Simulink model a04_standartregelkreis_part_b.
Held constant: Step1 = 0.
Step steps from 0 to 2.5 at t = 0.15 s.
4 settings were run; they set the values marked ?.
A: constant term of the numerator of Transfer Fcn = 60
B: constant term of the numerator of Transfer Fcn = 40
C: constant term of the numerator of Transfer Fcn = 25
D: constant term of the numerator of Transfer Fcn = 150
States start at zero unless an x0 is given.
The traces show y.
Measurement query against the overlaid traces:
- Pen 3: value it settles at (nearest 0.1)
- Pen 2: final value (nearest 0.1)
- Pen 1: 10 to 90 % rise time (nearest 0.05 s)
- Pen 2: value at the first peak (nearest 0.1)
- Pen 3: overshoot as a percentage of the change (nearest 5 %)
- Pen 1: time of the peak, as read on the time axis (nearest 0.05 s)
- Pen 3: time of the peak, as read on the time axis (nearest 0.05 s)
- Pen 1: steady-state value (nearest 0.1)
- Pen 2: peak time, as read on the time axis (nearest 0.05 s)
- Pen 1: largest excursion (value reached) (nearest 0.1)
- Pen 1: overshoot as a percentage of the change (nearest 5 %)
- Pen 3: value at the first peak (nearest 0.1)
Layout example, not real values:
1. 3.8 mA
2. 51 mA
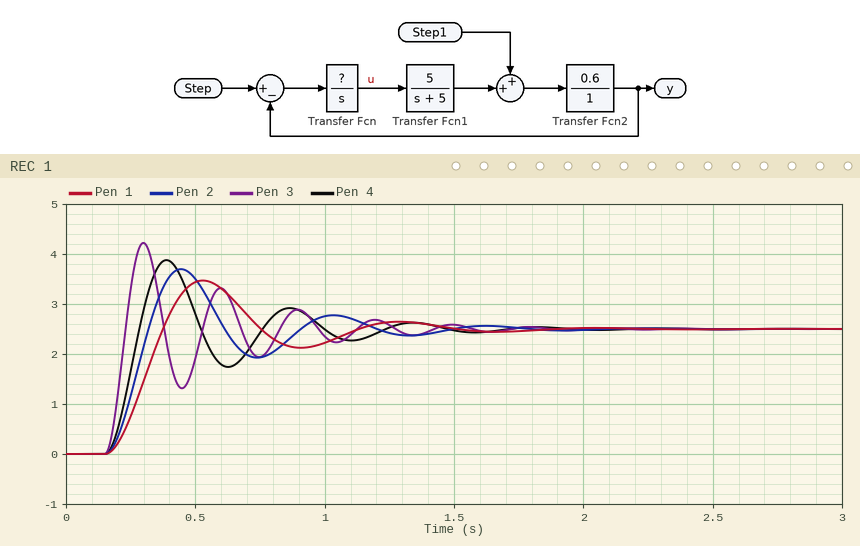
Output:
1. 2.5
2. 2.5
3. 0.15 s
4. 3.7
5. 70 %
6. 0.55 s
7. 0.30 s
8. 2.5
9. 0.45 s
10. 3.5
11. 40 %
12. 4.2
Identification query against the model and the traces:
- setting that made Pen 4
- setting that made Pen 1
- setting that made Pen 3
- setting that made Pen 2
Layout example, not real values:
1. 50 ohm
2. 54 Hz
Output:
1. A
2. C
3. D
4. B
